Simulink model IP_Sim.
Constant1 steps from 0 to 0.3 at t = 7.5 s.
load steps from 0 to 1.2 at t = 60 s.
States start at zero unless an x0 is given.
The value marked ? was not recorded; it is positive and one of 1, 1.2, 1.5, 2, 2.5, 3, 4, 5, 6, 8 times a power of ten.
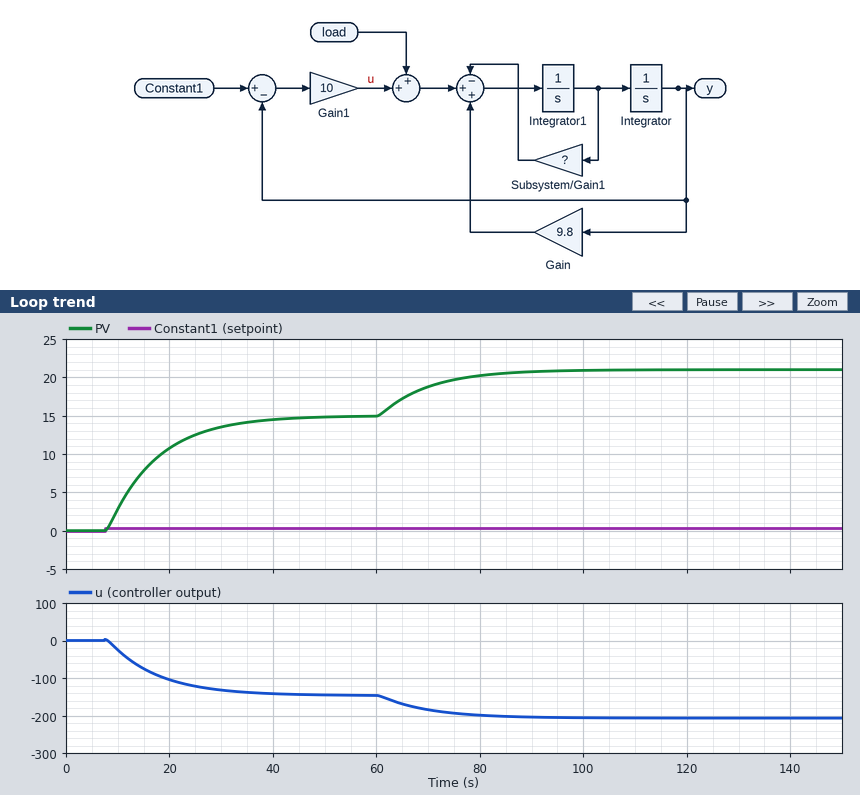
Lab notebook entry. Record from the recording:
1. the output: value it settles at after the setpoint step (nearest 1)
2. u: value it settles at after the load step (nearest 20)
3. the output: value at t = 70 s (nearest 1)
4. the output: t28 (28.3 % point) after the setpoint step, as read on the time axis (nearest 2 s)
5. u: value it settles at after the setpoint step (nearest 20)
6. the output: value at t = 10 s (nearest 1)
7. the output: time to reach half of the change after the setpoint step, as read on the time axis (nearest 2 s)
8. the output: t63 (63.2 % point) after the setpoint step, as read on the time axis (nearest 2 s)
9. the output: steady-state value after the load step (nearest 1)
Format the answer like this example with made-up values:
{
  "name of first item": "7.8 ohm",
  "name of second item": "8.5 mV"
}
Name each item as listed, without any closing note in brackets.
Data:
{
  "the output: value it settles at after the setpoint step": "15",
  "u: value it settles at after the load step": "-200",
  "the output: value at t = 70 s": "19",
  "the output: t28 (28.3 % point) after the setpoint step, as read on the time axis": "12 s",
  "u: value it settles at after the setpoint step": "-140",
  "the output: value at t = 10 s": "3",
  "the output: time to reach half of the change after the setpoint step, as read on the time axis": "14 s",
  "the output: t63 (63.2 % point) after the setpoint step, as read on the time axis": "18 s",
  "the output: steady-state value after the load step": "21"
}
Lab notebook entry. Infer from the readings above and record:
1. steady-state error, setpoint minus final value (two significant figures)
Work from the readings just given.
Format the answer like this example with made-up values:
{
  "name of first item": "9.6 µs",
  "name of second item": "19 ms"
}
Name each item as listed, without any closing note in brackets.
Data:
{
  "steady-state error, setpoint minus final value": "-15"
}
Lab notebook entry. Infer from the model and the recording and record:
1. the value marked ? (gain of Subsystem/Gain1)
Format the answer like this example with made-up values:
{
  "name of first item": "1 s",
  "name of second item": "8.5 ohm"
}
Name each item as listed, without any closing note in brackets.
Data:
{
  "the value marked ?": "2"
}
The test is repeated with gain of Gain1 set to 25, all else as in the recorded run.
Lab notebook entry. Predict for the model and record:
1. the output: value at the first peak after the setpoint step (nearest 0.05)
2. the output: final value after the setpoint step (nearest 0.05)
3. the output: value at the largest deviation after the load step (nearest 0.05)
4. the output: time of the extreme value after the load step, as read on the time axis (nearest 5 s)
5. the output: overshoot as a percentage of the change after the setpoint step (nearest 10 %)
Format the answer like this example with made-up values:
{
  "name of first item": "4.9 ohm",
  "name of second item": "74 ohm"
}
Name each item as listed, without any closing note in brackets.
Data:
{
  "the output: value at the first peak after the setpoint step": "0.70",
  "the output: final value after the setpoint step": "0.50",
  "the output: value at the largest deviation after the load step": "0.60",
  "the output: time of the extreme value after the load step, as read on the time axis": "60 s",
  "the output: overshoot as a percentage of the change after the setpoint step": "40 %"
}
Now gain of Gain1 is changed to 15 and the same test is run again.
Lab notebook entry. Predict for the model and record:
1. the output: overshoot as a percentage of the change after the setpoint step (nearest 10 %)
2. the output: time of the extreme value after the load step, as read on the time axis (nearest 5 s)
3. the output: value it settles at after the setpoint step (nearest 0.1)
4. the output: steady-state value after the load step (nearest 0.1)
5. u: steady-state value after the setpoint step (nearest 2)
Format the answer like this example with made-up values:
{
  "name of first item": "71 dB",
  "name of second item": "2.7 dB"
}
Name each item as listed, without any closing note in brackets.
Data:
{
  "the output: overshoot as a percentage of the change after the setpoint step": "20 %",
  "the output: time of the extreme value after the load step, as read on the time axis": "60 s",
  "the output: value it settles at after the setpoint step": "0.9",
  "the output: steady-state value after the load step": "1.1",
  "u: steady-state value after the setpoint step": "-8"
}
